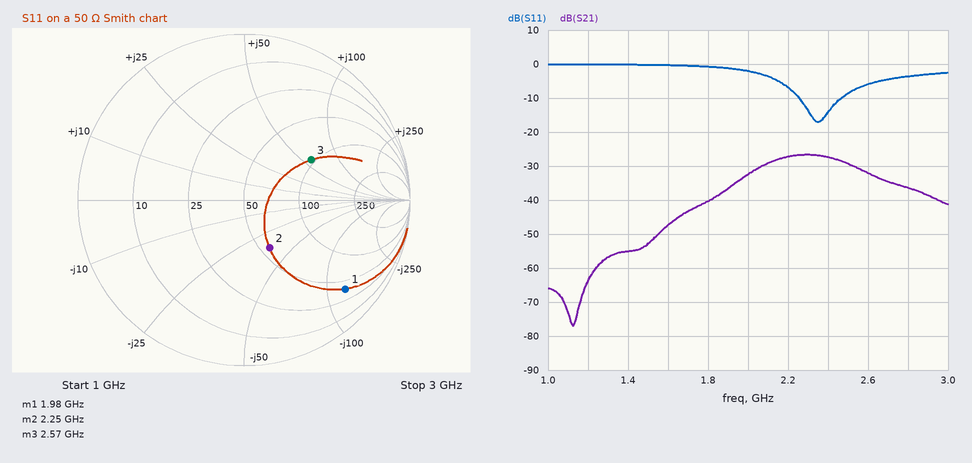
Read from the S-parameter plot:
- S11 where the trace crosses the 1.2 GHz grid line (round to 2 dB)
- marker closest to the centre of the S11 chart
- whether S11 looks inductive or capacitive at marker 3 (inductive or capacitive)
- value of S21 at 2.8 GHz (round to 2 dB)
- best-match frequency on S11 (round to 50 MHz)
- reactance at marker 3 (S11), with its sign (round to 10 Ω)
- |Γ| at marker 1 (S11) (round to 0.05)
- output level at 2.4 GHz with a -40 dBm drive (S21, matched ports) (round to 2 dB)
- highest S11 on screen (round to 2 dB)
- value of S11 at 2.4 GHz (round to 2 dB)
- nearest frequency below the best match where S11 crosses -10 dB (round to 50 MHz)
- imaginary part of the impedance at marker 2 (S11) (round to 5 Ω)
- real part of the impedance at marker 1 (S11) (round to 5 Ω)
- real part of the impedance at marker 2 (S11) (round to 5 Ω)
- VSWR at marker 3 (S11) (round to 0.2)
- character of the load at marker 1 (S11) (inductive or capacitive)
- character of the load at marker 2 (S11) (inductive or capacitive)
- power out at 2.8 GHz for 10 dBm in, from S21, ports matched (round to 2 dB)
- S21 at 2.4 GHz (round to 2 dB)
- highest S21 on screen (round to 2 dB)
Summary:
0 dB
marker 2
inductive
-36 dB
2.35 GHz
+60 Ω
0.80
-68 dBm
0 dB
-14 dB
2.25 GHz
-35 Ω
40 Ω
55 Ω
2.8
capacitive
capacitive
-26 dBm
-28 dB
-26 dB
